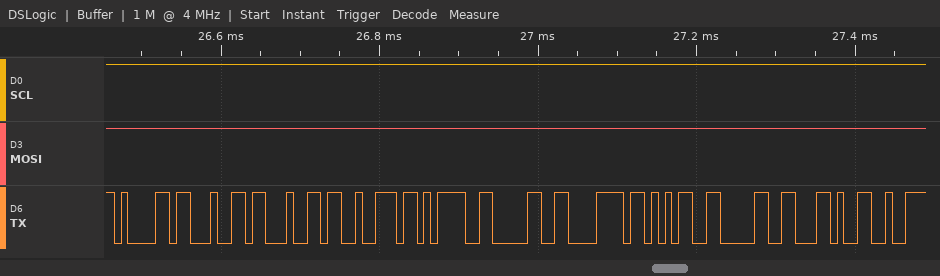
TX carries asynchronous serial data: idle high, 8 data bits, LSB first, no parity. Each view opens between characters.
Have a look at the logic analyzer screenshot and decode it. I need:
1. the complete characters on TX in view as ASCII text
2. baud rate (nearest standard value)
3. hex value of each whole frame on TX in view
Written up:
"addr=0x50,"
115200 baud
61, 64, 64, 72, 3D, 30, 78, 35, 30, 2C
